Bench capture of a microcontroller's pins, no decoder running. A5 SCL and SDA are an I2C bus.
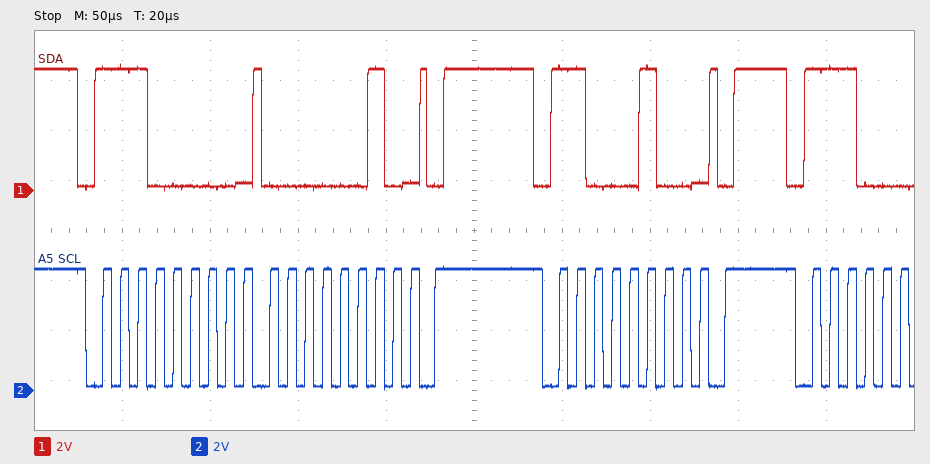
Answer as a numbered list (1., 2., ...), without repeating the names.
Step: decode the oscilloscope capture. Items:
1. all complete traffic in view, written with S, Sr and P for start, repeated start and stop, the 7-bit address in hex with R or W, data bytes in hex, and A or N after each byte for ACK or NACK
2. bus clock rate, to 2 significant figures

1. S 70W A 02 A P S 62W A P
2. 100 kHz
